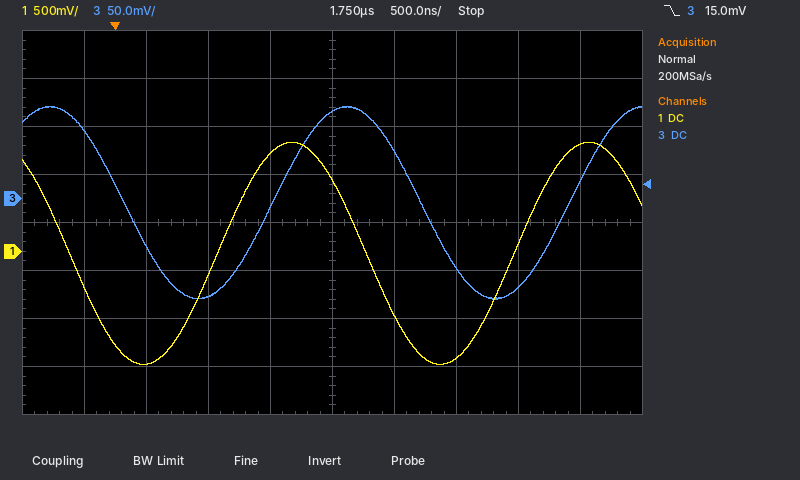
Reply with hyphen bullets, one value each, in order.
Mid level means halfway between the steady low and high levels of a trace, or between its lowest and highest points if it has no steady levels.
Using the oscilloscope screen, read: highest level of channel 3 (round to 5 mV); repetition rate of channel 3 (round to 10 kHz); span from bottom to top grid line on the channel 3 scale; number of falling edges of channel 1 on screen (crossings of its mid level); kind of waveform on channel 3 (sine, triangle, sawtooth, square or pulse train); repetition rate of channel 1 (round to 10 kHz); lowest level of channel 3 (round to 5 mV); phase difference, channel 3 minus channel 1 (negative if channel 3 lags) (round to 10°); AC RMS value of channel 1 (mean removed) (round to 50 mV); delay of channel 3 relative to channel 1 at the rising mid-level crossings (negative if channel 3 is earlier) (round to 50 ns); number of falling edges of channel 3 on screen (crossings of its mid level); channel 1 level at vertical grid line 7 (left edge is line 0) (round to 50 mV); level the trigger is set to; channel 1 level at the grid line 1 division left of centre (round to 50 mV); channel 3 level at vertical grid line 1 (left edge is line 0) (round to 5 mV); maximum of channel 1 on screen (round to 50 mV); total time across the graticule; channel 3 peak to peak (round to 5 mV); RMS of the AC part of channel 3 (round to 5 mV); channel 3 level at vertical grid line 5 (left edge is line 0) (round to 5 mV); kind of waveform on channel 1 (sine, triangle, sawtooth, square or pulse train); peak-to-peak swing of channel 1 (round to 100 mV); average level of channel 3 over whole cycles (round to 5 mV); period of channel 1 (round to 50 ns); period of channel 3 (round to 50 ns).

- 95 mV
- 420 kHz
- 400 mV
- 2
- sine
- 420 kHz
- -105 mV
- -70°
- 800 mV
- +450 ns
- 2
- -1.10 V
- 15.0 mV
- 1.00 V
- 70 mV
- 1.15 V
- 5 µs
- 200 mV
- 70 mV
- 90 mV
- sine
- 2.30 V
- -5 mV
- 2.40 µs
- 2.40 µs
